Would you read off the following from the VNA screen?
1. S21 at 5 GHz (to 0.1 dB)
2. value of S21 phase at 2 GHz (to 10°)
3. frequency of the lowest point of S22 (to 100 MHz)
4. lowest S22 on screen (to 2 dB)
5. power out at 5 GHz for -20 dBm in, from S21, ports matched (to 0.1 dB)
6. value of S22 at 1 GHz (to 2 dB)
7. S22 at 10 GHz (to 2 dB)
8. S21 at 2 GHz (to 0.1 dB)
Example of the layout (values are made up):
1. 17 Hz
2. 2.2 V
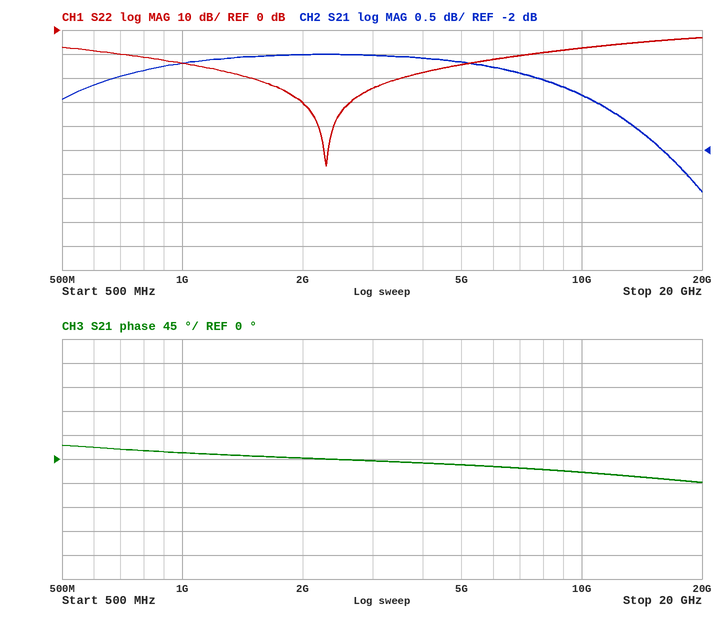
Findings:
1. -0.2 dB
2. 0°
3. 2.3 GHz
4. -56 dB
5. -20.2 dBm
6. -14 dB
7. -8 dB
8. 0.0 dB
